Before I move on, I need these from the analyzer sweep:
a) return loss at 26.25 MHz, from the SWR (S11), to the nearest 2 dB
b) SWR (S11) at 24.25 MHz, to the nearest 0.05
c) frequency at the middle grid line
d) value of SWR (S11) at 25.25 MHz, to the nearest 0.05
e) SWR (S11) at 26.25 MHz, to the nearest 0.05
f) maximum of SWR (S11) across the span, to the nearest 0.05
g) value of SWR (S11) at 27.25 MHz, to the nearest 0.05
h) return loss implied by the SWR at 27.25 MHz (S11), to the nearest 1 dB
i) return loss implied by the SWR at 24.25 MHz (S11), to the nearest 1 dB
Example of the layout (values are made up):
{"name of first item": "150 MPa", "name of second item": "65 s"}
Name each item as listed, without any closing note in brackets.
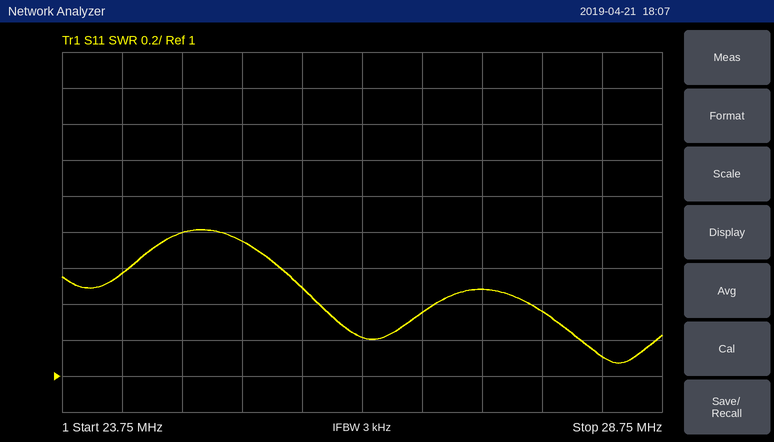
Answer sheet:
{"return loss at 26.25 MHz, from the SWR (S11), to the nearest 2 dB": "20 dB", "SWR (S11) at 24.25 MHz, to the nearest 0.05": "1.55", "frequency at the middle grid line": "26.25 MHz", "value of SWR (S11) at 25.25 MHz, to the nearest 0.05": "1.75", "SWR (S11) at 26.25 MHz, to the nearest 0.05": "1.20", "maximum of SWR (S11) across the span, to the nearest 0.05": "1.80", "value of SWR (S11) at 27.25 MHz, to the nearest 0.05": "1.50", "return loss implied by the SWR at 27.25 MHz (S11), to the nearest 1 dB": "14 dB", "return loss implied by the SWR at 24.25 MHz (S11), to the nearest 1 dB": "13 dB"}
